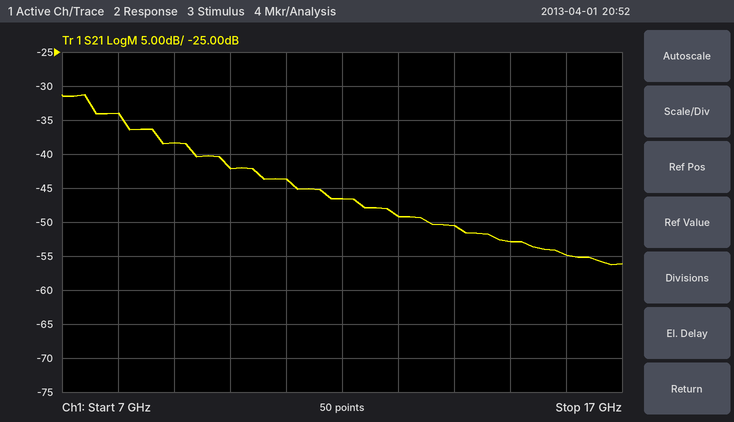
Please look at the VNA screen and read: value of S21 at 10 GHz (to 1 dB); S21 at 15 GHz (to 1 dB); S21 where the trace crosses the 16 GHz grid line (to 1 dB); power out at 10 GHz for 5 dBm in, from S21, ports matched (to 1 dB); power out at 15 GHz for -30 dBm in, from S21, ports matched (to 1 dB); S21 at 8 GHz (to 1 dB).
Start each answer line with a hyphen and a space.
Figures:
- -42 dB
- -53 dB
- -55 dB
- -37 dBm
- -83 dBm
- -34 dB
